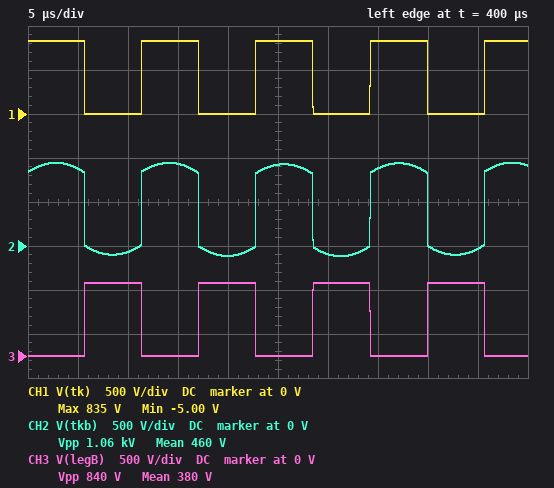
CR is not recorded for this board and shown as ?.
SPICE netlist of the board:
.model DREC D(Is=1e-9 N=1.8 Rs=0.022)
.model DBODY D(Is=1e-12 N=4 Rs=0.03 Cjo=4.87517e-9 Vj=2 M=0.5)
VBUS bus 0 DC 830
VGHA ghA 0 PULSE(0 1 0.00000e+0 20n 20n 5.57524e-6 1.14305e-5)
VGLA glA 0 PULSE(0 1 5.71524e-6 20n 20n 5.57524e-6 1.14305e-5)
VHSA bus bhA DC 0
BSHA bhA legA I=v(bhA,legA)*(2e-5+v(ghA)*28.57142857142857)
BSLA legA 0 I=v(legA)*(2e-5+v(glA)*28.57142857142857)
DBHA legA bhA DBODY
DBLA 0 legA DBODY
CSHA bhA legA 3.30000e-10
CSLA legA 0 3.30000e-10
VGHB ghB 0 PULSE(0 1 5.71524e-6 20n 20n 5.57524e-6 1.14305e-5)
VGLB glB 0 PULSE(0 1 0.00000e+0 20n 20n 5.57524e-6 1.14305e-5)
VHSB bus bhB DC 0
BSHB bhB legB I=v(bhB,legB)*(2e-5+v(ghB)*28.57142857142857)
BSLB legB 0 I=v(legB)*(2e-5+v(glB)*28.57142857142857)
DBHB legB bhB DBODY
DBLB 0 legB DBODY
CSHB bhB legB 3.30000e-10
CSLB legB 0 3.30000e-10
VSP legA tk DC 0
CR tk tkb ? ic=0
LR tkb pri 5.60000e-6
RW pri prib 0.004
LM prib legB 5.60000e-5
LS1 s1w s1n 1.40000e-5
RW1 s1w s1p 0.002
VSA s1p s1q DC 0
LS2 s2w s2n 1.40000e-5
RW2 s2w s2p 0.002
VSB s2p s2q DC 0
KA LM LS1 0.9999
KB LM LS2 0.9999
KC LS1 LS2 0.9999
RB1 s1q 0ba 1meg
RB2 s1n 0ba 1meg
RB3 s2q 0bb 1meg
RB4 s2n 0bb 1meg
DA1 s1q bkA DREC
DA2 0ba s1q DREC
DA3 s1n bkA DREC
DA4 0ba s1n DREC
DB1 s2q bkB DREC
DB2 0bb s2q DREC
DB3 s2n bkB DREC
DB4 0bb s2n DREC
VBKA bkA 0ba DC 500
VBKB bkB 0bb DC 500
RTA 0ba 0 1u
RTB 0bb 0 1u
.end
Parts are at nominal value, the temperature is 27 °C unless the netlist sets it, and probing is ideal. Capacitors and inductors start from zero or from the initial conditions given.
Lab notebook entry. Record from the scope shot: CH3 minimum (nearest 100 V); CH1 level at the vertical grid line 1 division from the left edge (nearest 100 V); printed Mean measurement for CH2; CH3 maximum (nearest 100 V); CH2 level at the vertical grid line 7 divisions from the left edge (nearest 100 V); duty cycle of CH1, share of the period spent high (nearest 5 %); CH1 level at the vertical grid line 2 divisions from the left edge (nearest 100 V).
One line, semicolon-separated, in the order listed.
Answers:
0 V; 800 V; 460 V; 800 V; 900 V; 50 %; 0 V
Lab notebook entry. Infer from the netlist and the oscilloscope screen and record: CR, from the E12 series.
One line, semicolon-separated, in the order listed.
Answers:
560 nF
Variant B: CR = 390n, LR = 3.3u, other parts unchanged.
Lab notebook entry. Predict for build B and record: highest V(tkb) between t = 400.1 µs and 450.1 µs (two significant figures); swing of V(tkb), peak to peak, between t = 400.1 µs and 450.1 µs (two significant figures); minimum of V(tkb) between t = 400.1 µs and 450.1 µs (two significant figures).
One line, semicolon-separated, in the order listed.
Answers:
1.0 kV; 1.2 kV; -190 V
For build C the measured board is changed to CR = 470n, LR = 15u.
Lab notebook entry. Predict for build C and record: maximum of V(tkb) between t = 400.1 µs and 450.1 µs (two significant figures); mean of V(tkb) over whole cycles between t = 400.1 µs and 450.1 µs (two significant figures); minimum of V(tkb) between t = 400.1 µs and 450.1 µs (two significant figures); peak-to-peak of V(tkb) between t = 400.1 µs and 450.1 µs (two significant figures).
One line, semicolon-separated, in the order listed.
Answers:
1.1 kV; 390 V; -280 V; 1.4 kV
